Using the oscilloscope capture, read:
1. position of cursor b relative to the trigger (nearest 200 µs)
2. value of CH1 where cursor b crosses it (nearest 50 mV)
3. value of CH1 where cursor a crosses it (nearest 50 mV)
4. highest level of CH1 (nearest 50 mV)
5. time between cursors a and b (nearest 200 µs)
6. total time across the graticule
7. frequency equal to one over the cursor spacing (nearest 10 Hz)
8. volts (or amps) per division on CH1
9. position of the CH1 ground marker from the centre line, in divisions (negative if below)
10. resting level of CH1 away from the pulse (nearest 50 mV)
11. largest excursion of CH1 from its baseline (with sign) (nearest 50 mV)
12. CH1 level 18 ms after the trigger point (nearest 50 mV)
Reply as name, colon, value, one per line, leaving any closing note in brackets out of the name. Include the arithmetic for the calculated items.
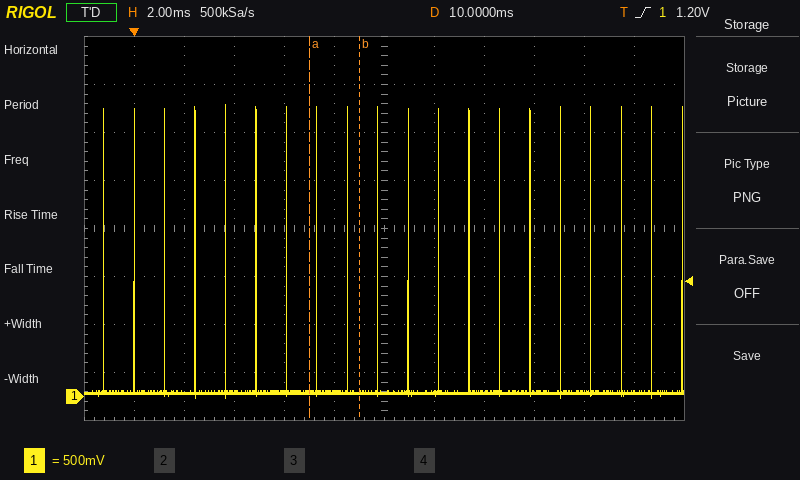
position of cursor b relative to the trigger: +9.0 ms
value of CH1 where cursor b crosses it: 50 mV
value of CH1 where cursor a crosses it: 50 mV
highest level of CH1: 3.05 V
time between cursors a and b: 2.0 ms
total time across the graticule: 24 ms
frequency equal to one over the cursor spacing: 1 / 2.0 ms ≈ 500 Hz
volts (or amps) per division on CH1: 500 mV
position of the CH1 ground marker from the centre line, in divisions: -3.5 div
resting level of CH1 away from the pulse: 50 mV
largest excursion of CH1 from its baseline (with sign): 3.05 V − (50 mV) = +3.00 V
CH1 level 18 ms after the trigger point: 50 mV
